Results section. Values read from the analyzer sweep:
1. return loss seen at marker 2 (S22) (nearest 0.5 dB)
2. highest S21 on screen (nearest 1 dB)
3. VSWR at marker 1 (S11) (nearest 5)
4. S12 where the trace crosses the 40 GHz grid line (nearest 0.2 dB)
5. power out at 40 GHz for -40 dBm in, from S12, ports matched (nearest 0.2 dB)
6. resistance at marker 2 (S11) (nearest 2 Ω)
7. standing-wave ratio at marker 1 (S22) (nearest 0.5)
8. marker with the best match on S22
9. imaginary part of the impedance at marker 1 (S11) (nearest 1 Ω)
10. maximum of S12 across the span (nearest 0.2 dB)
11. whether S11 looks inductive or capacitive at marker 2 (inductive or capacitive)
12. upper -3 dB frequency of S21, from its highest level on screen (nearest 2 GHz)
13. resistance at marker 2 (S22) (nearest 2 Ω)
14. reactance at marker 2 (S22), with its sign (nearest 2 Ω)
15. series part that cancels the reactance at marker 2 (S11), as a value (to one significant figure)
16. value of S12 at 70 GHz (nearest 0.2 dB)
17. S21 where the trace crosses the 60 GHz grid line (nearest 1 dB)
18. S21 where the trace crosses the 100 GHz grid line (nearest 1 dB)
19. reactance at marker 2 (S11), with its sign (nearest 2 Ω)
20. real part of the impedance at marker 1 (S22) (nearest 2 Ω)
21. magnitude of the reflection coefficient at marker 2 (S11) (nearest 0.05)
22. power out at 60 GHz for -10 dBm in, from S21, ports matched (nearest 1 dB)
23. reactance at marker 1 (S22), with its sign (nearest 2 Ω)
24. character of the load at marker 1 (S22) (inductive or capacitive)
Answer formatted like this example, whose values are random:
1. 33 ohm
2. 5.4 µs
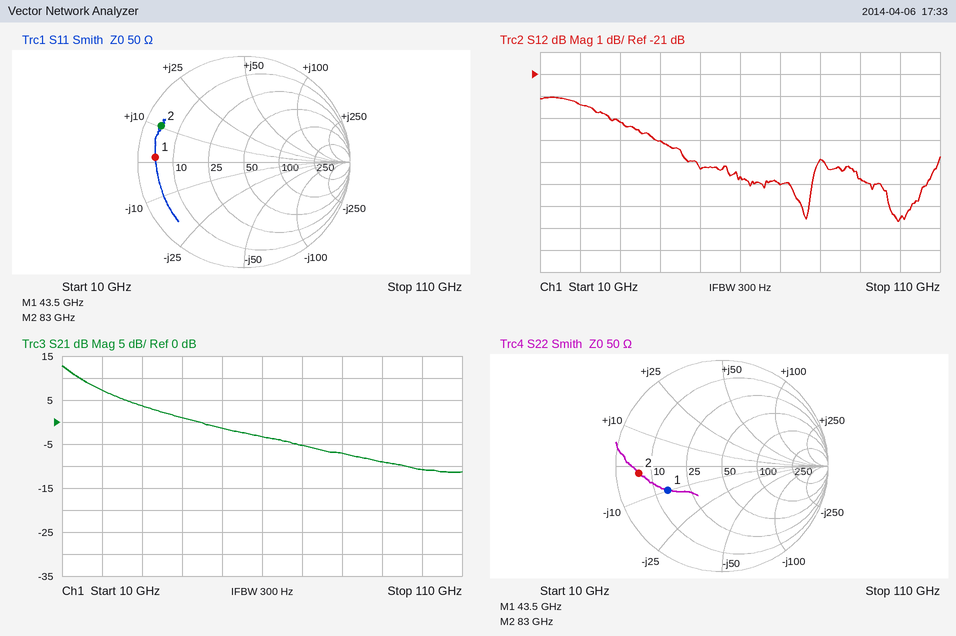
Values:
1. 2.0 dB
2. 13 dB
3. 10
4. -24.0 dB
5. -64.0 dBm
6. 4 Ω
7. 3.5
8. marker 1
9. +1 Ω
10. -22.0 dB
11. inductive
12. 14 GHz
13. 6 Ω
14. -2 Ω
15. 200 fF
16. -26.0 dB
17. -3 dB
18. -11 dB
19. +10 Ω
20. 14 Ω
21. 0.85
22. -13 dBm
23. -10 Ω
24. capacitive
